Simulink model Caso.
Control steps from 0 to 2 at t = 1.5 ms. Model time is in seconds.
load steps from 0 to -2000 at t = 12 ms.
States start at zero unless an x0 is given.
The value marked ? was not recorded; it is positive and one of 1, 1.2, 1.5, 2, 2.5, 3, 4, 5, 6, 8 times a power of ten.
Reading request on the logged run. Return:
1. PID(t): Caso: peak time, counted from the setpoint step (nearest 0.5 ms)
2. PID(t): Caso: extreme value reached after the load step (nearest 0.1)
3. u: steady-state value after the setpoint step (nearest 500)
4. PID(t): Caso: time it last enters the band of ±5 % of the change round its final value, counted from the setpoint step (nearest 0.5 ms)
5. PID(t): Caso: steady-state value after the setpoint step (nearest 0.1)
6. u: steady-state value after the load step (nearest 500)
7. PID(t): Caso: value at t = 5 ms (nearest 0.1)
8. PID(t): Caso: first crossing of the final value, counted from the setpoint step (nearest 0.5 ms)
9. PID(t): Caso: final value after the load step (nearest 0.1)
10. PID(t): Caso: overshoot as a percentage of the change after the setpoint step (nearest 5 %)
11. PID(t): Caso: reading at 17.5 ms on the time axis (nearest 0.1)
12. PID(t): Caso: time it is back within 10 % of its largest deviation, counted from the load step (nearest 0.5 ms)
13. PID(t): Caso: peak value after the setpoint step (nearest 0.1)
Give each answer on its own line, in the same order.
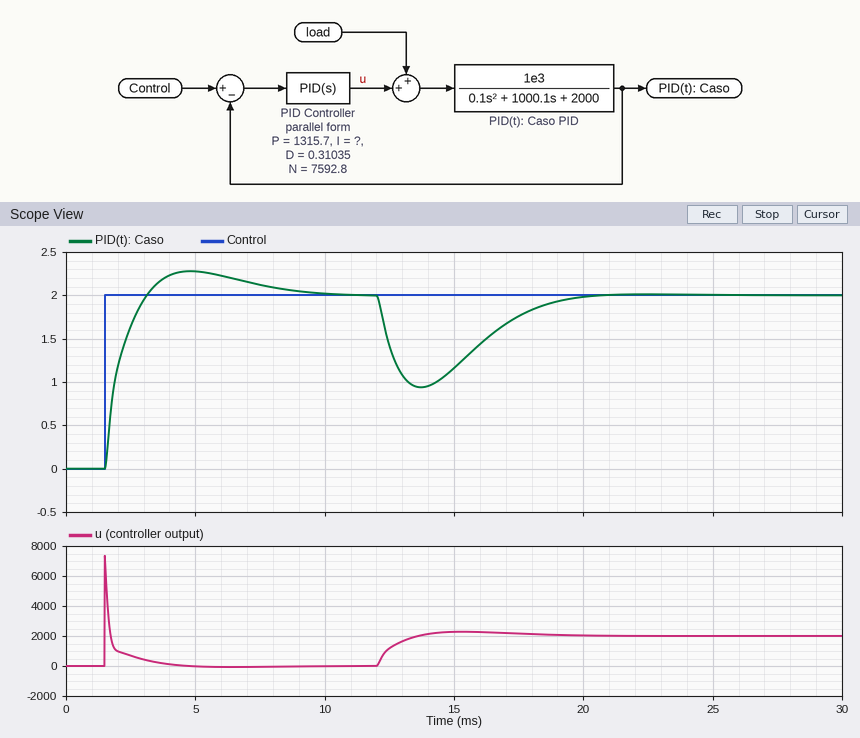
3.5 ms
0.9
0
6.5 ms
2.0
2000
2.3
1.5 ms
2.0
15 %
1.8
6.5 ms
2.3
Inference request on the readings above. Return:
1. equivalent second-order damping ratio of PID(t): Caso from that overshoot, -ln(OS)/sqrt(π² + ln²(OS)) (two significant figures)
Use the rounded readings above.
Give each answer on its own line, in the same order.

0.52
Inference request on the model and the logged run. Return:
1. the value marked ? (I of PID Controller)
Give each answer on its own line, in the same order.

500000
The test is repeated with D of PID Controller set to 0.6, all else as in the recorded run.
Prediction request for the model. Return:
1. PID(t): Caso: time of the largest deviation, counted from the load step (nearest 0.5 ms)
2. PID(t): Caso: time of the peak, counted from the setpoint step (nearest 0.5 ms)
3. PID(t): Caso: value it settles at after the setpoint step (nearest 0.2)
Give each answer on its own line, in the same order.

2.0 ms
4.0 ms
2.0
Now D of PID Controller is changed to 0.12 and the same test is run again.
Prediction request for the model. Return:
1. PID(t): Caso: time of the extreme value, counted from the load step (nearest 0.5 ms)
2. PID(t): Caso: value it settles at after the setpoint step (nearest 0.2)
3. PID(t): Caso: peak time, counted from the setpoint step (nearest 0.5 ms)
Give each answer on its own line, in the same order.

1.5 ms
2.0
3.0 ms
